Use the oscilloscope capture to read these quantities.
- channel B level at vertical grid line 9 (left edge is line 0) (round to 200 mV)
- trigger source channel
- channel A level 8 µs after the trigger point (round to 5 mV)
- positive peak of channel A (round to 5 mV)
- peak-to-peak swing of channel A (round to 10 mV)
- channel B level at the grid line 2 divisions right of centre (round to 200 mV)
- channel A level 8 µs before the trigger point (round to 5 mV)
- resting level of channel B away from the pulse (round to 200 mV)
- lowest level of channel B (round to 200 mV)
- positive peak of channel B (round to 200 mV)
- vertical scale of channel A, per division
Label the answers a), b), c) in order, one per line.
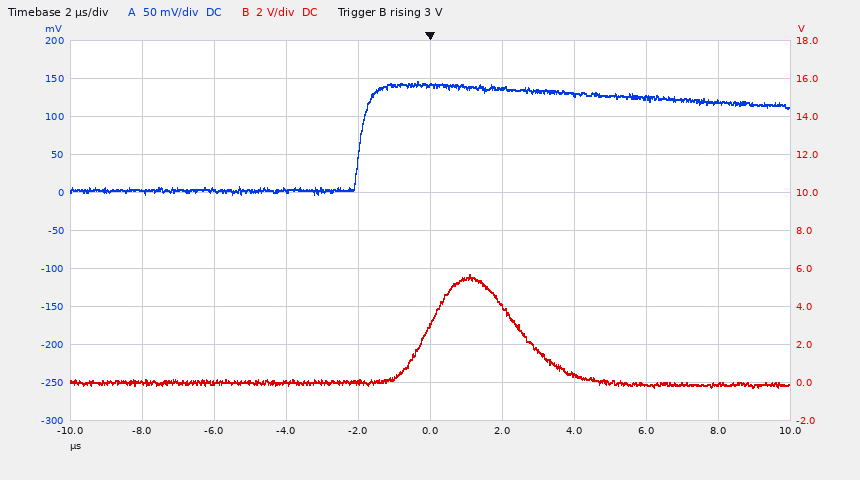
a) 0.0 V
b) channel B
c) 120 mV
d) 145 mV
e) 150 mV
f) 400 mV
g) 0 mV
h) 0.0 V
i) -200 mV
j) 5.6 V
k) 50 mV
